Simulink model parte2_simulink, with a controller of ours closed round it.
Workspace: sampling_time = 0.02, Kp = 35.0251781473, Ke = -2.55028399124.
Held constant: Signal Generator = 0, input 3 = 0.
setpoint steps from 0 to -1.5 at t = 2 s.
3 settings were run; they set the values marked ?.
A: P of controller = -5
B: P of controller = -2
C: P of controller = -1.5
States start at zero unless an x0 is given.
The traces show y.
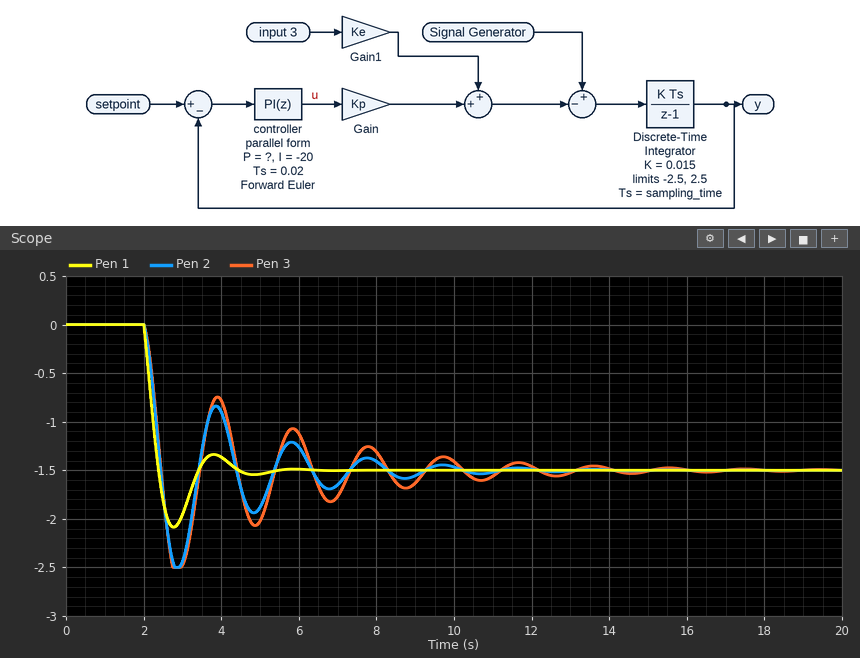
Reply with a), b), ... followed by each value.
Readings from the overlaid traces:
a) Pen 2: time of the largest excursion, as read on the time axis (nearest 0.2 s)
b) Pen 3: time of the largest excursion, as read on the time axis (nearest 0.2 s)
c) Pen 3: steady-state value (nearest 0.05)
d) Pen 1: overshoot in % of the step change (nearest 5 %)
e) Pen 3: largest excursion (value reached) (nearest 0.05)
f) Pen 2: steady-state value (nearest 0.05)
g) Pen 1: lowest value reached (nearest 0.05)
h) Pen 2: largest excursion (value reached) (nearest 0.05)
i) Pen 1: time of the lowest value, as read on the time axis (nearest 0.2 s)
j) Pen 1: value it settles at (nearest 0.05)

a) 2.8 s
b) 2.8 s
c) -1.50
d) 40 %
e) -2.50
f) -1.50
g) -2.10
h) -2.50
i) 2.8 s
j) -1.50
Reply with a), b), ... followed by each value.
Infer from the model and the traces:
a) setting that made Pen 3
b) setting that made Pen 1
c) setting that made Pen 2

a) C
b) A
c) B
